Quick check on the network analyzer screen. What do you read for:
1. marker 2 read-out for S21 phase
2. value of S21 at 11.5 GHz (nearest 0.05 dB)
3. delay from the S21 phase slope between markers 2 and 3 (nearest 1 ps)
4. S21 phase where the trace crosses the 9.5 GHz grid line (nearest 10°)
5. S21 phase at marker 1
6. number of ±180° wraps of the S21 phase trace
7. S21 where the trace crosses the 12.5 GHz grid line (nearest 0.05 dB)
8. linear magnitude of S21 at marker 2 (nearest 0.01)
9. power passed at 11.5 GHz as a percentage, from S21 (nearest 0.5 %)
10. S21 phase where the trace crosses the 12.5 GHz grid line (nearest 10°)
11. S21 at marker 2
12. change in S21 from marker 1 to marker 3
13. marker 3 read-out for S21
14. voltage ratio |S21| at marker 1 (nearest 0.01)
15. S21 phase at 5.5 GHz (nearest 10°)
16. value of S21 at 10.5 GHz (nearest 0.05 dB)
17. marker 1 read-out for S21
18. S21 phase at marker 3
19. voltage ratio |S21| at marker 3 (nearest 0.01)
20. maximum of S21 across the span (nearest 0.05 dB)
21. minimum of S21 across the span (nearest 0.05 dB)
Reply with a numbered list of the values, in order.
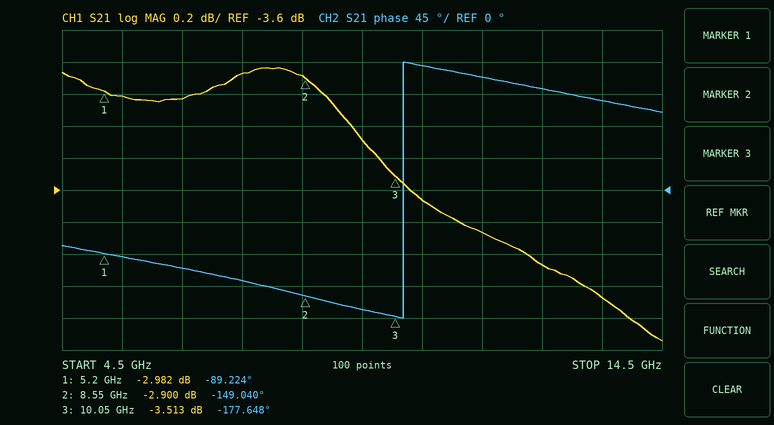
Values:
1. -149.040°
2. -3.85 dB
3. 53 ps
4. -170°
5. -89.224°
6. 1
7. -4.05 dB
8. 0.72
9. 41.0 %
10. 140°
11. -2.900 dB
12. -0.531 dB
13. -3.513 dB
14. 0.71
15. -90°
16. -3.65 dB
17. -2.982 dB
18. -177.648°
19. 0.67
20. -2.85 dB
21. -4.55 dB
